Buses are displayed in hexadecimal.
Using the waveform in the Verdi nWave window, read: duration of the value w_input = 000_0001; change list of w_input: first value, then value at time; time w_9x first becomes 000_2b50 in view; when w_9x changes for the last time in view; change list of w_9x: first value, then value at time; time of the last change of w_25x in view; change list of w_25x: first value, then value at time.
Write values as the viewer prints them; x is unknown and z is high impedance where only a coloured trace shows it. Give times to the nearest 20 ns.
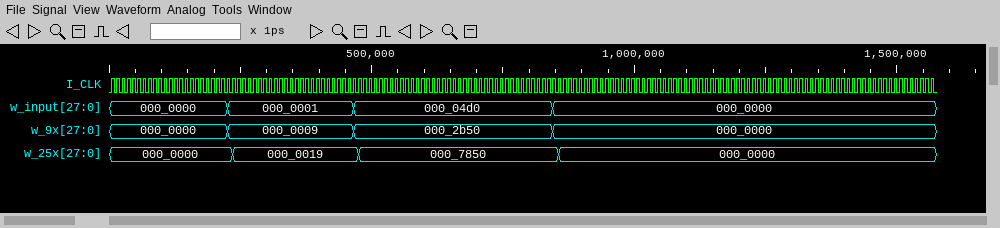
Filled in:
240 ns
000_0000, 000_0001 at 220 ns, 000_04d0 at 460 ns, 000_0000 at 840 ns
460 ns
840 ns
000_0000, 000_0009 at 220 ns, 000_2b50 at 460 ns, 000_0000 at 840 ns
860 ns
000_0000, 000_0019 at 240 ns, 000_7850 at 480 ns, 000_0000 at 860 ns
